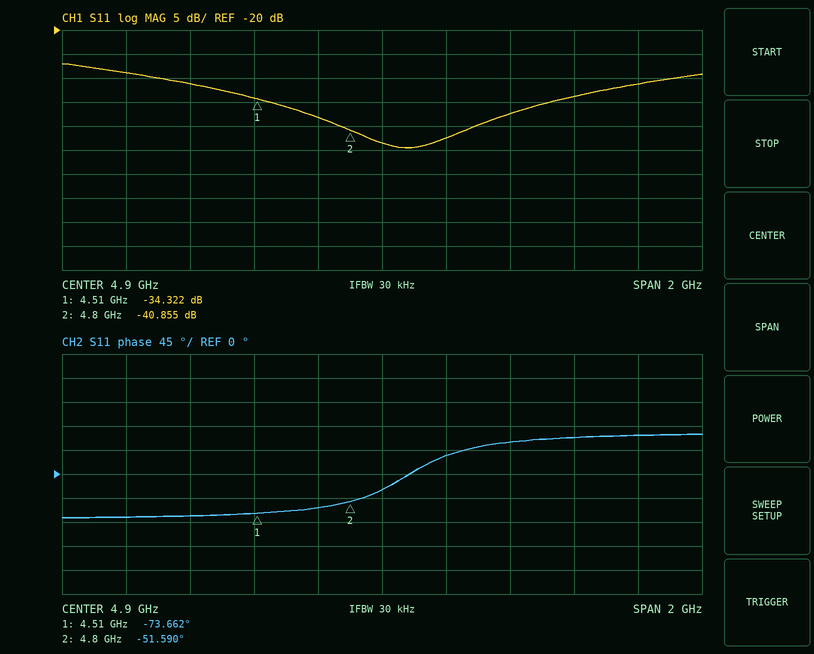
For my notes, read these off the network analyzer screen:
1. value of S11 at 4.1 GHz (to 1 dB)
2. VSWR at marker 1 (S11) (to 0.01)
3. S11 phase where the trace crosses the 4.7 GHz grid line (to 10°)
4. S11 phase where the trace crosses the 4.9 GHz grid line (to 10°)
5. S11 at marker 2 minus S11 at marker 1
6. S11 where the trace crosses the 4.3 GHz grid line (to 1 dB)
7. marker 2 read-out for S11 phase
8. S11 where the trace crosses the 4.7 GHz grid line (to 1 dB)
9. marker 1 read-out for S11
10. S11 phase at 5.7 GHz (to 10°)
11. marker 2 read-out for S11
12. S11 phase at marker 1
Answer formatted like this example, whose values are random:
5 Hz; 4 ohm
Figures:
-29 dB; 1.04; -60°; -30°; -6.533 dB; -31 dB; -51.590°; -38 dB; -34.322 dB; 70°; -40.855 dB; -73.662°
